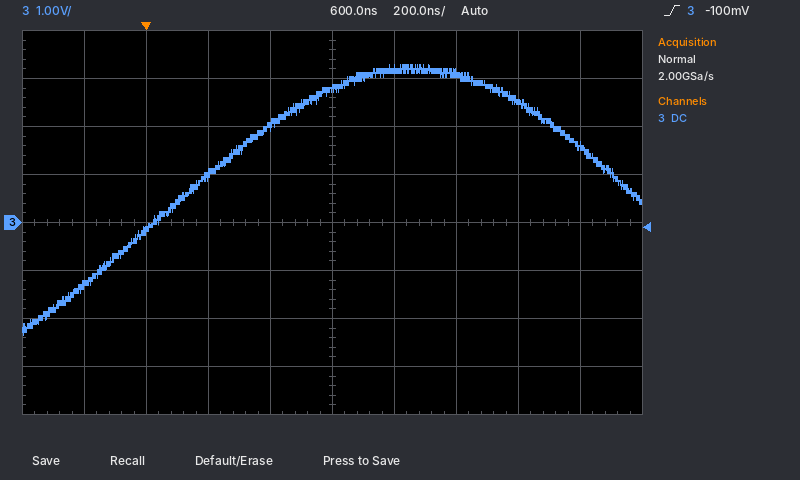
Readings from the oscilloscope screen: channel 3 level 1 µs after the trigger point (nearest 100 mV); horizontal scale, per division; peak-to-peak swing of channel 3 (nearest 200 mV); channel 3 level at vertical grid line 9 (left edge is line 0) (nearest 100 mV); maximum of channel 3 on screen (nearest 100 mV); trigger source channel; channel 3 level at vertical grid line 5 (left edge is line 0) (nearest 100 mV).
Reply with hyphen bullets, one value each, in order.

- 3.1 V
- 200 ns
- 5.6 V
- 1.6 V
- 3.3 V
- channel 3
- 2.8 V
